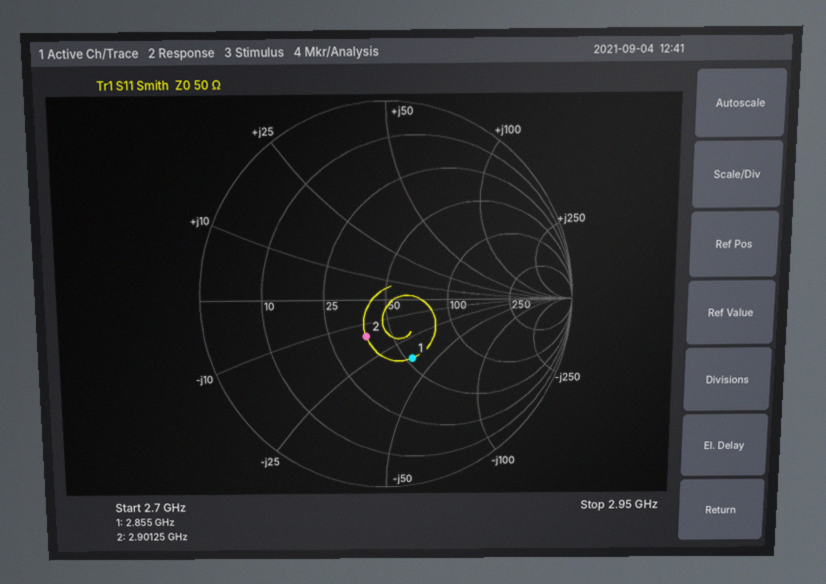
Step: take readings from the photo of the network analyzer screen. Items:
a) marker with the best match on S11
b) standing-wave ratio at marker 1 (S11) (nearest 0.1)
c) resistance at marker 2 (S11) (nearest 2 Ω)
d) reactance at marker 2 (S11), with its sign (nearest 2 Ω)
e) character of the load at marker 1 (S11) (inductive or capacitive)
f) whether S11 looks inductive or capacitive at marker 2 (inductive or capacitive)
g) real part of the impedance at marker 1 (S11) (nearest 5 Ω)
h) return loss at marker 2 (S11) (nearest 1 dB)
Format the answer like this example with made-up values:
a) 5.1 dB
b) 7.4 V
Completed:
a) marker 2
b) 2.0
c) 38 Ω
d) -16 Ω
e) capacitive
f) capacitive
g) 55 Ω
h) 13 dB
